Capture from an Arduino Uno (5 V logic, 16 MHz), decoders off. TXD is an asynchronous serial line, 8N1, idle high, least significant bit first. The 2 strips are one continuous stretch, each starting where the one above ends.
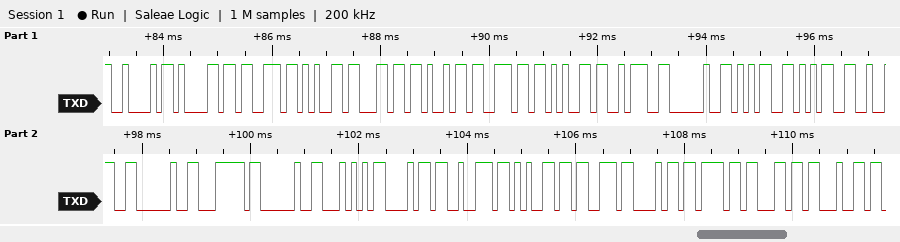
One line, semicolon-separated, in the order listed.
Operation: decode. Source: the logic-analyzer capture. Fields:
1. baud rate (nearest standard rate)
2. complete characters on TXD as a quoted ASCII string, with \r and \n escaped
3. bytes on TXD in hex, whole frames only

9600 baud; "Baseline: 552 | Threshold"; 42 61 73 65 6C 69 6E 65 3A 20 35 35 32 20 7C 20 54 68 72 65 73 68 6F 6C 64
